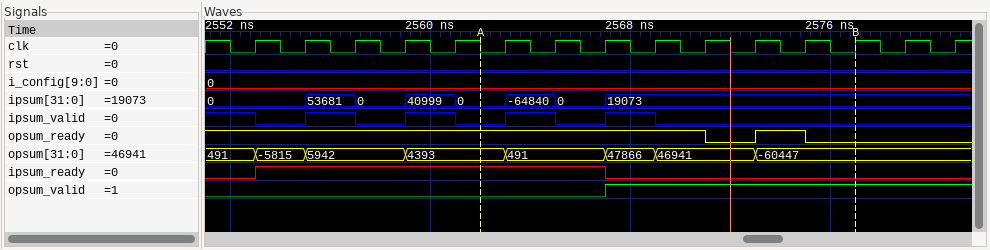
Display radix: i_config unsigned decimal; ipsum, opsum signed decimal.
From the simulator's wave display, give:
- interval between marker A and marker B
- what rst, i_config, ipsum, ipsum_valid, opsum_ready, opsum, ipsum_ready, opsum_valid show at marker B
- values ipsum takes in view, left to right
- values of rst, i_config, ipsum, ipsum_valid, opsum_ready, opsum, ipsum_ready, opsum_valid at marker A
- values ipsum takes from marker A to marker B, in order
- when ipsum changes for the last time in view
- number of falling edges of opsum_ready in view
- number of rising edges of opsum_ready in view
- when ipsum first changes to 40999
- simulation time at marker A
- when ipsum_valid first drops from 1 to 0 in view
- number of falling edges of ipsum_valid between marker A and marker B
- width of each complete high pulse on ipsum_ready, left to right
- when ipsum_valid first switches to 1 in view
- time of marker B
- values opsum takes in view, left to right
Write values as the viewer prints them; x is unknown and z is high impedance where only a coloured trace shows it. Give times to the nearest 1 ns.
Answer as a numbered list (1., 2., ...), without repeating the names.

1. 15 ns
2. rst=0, i_config=0, ipsum=19073, ipsum_valid=0, opsum_ready=0, opsum=-60447, ipsum_ready=0, opsum_valid=1
3. 0, 53681, 0, 40999, 0, -64840, 0, 19073
4. rst=0, i_config=0, ipsum=0, ipsum_valid=0, opsum_ready=1, opsum=4393, ipsum_ready=1, opsum_valid=0
5. 0, -64840, 0, 19073
6. 2567 ns
7. 2
8. 1
9. 2559 ns
10. 2562 ns
11. 2553 ns
12. 2
13. 14 ns
14. 2555 ns
15. 2577 ns
16. 491, -5815, 5942, 4393, 491, 47866, 46941, -60447
